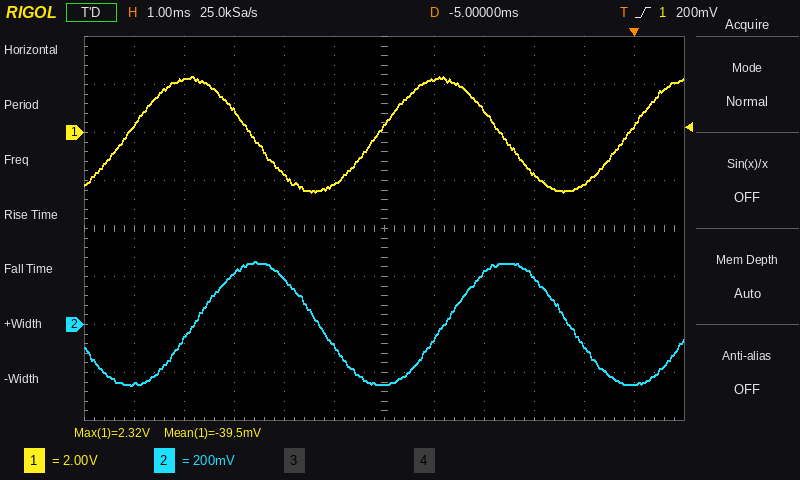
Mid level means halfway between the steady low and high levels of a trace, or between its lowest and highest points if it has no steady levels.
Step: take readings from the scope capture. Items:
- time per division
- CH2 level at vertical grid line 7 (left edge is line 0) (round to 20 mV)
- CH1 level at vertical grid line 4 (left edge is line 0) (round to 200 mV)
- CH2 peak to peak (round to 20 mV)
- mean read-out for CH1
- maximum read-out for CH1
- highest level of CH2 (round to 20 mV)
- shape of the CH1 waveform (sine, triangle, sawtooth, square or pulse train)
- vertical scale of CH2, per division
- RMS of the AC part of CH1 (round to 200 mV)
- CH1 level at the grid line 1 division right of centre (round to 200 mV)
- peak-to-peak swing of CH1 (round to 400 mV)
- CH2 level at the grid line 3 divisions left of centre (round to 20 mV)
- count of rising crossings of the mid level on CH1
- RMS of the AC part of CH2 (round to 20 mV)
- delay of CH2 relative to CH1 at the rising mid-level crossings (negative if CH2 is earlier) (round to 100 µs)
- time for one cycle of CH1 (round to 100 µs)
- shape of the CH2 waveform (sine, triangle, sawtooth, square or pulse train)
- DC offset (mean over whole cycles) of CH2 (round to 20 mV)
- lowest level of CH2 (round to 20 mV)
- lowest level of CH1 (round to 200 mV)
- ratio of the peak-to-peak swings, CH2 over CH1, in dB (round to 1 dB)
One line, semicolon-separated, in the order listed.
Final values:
1 ms; -60 mV; -1.8 V; 520 mV; -39.5 mV; 2.32 V; 260 mV; sine; 200 mV; 1.6 V; 2.2 V; 4.8 V; 220 mV; 3; 180 mV; +1.4 ms; 5.0 ms; sine; 0 mV; -260 mV; -2.4 V; -19 dB
